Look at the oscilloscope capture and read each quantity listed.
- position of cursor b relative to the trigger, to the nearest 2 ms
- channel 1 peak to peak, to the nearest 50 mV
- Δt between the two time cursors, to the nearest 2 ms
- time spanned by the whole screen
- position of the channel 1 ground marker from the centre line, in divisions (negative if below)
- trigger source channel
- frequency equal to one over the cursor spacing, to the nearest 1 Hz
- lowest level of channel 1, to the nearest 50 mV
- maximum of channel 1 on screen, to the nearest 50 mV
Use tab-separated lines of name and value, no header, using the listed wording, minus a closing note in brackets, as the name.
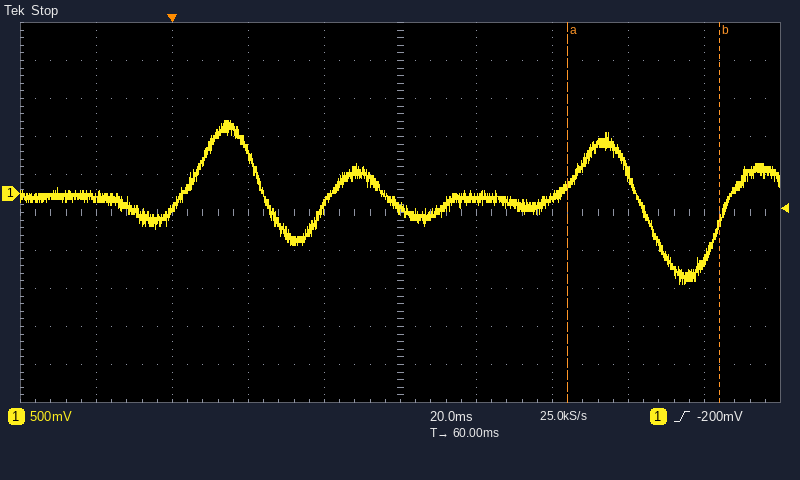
position of cursor b relative to the trigger, to the nearest 2 ms	+144 ms
channel 1 peak to peak, to the nearest 50 mV	2.15 V
Δt between the two time cursors, to the nearest 2 ms	40 ms
time spanned by the whole screen	200 ms
position of the channel 1 ground marker from the centre line, in divisions	+0.5 div
trigger source channel	channel 1
frequency equal to one over the cursor spacing, to the nearest 1 Hz	25 Hz
lowest level of channel 1, to the nearest 50 mV	-1.20 V
maximum of channel 1 on screen, to the nearest 50 mV	950 mV
